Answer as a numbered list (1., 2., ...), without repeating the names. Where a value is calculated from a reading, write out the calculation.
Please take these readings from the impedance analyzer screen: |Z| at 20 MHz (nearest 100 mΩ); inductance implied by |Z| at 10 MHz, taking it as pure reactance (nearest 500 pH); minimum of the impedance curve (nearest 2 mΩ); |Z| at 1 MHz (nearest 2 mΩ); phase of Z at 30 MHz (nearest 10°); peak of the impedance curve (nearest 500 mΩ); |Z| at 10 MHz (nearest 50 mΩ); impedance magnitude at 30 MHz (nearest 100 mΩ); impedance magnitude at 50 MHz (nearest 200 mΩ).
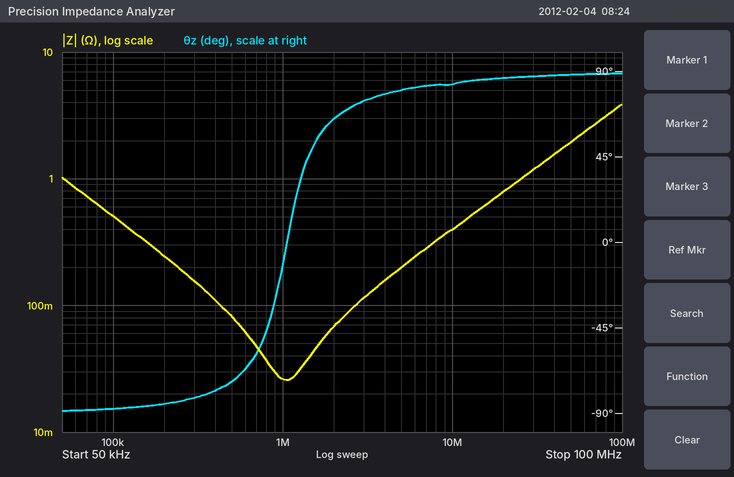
1. 800 mΩ
2. L = 400 mΩ/(2π × 10 MHz) ≈ 6.37 nH, so 6.5 nH to the nearest 500 pH
3. 26 mΩ
4. 26 mΩ
5. 90°
6. 4.0 Ω
7. 400 mΩ
8. 1.2 Ω
9. 2.0 Ω
